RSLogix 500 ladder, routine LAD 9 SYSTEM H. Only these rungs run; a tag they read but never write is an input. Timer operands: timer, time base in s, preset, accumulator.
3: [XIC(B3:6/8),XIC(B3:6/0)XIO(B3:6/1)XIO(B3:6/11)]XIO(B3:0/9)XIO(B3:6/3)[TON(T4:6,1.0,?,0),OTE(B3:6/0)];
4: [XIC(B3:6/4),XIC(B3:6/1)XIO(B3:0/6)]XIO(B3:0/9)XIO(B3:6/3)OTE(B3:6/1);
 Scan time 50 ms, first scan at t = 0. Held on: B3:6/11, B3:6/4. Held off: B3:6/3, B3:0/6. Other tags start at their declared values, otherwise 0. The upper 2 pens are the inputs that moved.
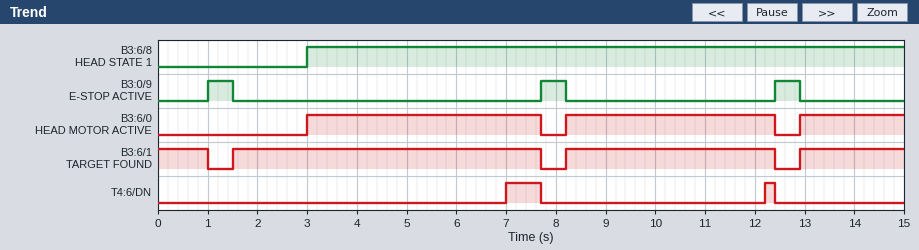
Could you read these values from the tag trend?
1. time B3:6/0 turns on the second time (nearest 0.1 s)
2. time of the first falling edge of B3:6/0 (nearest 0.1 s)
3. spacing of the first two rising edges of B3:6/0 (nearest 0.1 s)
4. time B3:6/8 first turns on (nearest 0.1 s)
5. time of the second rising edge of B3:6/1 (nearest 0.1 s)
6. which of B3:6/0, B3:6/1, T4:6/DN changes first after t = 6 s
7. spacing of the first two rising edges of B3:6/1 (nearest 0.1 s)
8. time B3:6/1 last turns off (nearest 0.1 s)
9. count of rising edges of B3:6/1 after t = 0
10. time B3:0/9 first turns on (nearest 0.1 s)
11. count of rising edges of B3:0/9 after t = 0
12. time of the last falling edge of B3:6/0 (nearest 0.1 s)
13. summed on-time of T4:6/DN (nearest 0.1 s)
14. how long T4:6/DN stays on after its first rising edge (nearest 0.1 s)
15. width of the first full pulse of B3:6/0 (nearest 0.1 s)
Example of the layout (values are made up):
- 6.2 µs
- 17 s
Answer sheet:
- 8.2 s
- 7.7 s
- 5.2 s
- 3.0 s
- 8.2 s
- T4:6/DN
- 6.7 s
- 12.4 s
- 3
- 1.0 s
- 3
- 12.4 s
- 0.9 s
- 0.7 s
- 4.7 s
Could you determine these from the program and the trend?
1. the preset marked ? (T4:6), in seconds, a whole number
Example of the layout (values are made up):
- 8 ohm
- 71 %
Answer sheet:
- 4 s
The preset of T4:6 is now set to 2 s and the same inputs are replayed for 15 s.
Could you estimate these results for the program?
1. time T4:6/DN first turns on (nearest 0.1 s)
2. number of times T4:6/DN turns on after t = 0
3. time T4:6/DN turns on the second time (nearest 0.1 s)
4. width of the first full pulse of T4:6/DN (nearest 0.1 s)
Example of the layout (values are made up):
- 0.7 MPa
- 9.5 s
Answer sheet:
- 5.0 s
- 3
- 10.2 s
- 2.7 s
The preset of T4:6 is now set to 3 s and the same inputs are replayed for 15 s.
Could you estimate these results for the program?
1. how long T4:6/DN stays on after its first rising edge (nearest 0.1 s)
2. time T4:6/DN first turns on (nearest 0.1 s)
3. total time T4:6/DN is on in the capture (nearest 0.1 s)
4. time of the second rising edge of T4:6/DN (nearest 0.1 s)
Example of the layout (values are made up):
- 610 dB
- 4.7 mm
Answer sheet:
- 1.7 s
- 6.0 s
- 2.9 s
- 11.2 s
